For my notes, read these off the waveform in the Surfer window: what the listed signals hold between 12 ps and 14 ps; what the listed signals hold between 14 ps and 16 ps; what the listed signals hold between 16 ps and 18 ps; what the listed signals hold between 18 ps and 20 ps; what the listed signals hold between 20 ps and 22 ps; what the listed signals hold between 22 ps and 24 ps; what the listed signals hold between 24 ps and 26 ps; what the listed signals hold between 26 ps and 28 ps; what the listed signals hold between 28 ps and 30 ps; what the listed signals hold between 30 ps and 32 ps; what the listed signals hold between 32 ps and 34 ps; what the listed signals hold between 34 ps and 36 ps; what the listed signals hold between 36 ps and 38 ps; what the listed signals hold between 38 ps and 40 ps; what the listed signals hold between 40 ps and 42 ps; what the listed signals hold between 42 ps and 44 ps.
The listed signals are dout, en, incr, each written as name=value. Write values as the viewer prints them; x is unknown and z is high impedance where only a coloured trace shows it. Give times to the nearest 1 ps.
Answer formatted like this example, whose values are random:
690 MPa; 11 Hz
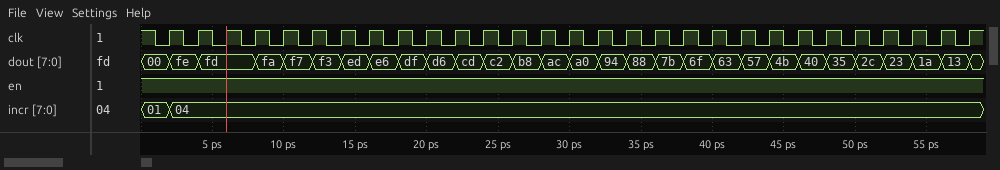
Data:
dout=f3, en=1, incr=04; dout=ed, en=1, incr=04; dout=e6, en=1, incr=04; dout=df, en=1, incr=04; dout=d6, en=1, incr=04; dout=cd, en=1, incr=04; dout=c2, en=1, incr=04; dout=b8, en=1, incr=04; dout=ac, en=1, incr=04; dout=a0, en=1, incr=04; dout=94, en=1, incr=04; dout=88, en=1, incr=04; dout=7b, en=1, incr=04; dout=6f, en=1, incr=04; dout=63, en=1, incr=04; dout=57, en=1, incr=04
